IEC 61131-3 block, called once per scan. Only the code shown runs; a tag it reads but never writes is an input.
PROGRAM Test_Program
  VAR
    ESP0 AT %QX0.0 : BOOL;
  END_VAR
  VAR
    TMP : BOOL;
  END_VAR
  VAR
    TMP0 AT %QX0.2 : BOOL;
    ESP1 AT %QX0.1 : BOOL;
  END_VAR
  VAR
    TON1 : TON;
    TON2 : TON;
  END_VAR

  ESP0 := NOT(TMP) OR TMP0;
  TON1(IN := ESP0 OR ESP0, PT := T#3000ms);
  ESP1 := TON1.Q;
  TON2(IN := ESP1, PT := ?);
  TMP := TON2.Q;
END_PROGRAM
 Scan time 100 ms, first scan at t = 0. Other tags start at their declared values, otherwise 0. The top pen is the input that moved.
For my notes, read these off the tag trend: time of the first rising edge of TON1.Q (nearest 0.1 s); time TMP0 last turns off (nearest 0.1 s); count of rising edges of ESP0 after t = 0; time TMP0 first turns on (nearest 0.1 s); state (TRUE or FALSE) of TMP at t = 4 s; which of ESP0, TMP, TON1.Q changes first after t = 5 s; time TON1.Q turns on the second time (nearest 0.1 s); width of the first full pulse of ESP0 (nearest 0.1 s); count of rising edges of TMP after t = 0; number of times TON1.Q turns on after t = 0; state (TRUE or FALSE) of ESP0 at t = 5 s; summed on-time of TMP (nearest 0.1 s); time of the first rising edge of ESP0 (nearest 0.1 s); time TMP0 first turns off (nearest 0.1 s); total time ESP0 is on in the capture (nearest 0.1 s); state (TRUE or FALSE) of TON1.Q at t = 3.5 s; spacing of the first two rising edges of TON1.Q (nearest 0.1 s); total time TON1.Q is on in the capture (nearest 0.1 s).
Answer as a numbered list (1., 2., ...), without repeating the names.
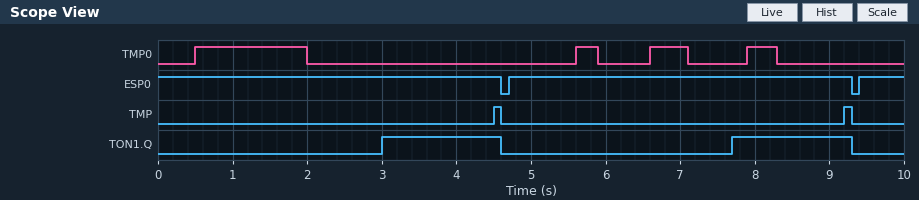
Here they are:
1. 3.0 s
2. 8.3 s
3. 2
4. 0.5 s
5. FALSE
6. TON1.Q
7. 7.7 s
8. 4.6 s
9. 2
10. 2
11. TRUE
12. 0.2 s
13. 4.7 s
14. 2.0 s
15. 9.8 s
16. TRUE
17. 4.7 s
18. 3.2 s
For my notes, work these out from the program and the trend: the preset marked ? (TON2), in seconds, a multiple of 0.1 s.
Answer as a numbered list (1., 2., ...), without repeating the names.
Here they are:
1. 1.5 s
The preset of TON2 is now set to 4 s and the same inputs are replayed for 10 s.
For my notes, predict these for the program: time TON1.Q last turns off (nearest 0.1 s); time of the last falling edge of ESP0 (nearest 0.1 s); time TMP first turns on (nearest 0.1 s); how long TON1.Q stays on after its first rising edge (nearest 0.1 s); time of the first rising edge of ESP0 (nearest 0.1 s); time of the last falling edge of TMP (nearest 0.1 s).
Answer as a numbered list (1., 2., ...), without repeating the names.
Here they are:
1. 7.1 s
2. 7.1 s
3. 7.0 s
4. 4.1 s
5. 7.2 s
6. 7.1 s
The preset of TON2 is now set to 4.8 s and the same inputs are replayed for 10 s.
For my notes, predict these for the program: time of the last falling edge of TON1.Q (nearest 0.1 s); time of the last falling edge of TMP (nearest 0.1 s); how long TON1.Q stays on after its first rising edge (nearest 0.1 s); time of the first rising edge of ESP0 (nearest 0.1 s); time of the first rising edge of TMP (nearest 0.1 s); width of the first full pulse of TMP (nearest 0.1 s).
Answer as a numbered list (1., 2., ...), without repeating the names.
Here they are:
1. 8.3 s
2. 8.3 s
3. 5.3 s
4. 8.4 s
5. 7.8 s
6. 0.5 s
